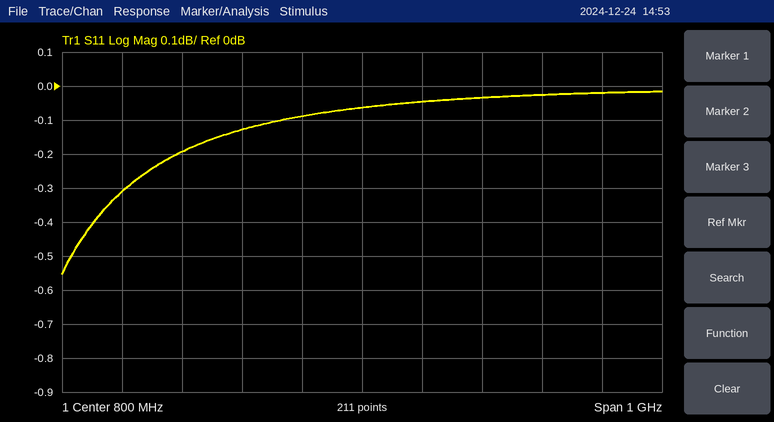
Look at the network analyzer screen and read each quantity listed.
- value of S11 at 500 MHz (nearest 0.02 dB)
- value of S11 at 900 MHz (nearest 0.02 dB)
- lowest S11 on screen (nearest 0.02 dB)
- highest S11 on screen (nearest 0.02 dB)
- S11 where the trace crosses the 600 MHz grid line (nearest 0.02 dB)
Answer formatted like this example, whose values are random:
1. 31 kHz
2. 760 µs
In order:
1. -0.20 dB
2. -0.04 dB
3. -0.56 dB
4. -0.02 dB
5. -0.12 dB
